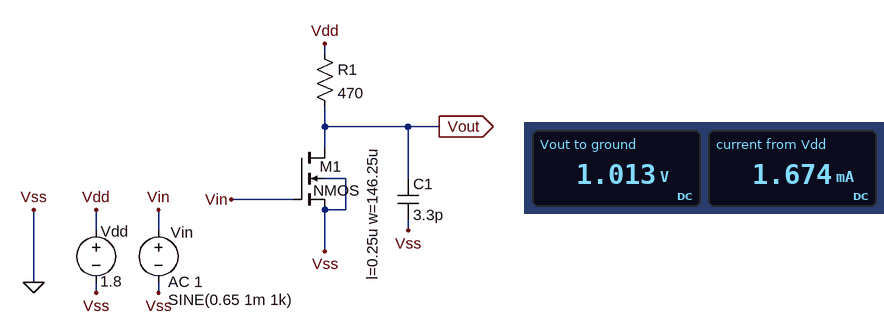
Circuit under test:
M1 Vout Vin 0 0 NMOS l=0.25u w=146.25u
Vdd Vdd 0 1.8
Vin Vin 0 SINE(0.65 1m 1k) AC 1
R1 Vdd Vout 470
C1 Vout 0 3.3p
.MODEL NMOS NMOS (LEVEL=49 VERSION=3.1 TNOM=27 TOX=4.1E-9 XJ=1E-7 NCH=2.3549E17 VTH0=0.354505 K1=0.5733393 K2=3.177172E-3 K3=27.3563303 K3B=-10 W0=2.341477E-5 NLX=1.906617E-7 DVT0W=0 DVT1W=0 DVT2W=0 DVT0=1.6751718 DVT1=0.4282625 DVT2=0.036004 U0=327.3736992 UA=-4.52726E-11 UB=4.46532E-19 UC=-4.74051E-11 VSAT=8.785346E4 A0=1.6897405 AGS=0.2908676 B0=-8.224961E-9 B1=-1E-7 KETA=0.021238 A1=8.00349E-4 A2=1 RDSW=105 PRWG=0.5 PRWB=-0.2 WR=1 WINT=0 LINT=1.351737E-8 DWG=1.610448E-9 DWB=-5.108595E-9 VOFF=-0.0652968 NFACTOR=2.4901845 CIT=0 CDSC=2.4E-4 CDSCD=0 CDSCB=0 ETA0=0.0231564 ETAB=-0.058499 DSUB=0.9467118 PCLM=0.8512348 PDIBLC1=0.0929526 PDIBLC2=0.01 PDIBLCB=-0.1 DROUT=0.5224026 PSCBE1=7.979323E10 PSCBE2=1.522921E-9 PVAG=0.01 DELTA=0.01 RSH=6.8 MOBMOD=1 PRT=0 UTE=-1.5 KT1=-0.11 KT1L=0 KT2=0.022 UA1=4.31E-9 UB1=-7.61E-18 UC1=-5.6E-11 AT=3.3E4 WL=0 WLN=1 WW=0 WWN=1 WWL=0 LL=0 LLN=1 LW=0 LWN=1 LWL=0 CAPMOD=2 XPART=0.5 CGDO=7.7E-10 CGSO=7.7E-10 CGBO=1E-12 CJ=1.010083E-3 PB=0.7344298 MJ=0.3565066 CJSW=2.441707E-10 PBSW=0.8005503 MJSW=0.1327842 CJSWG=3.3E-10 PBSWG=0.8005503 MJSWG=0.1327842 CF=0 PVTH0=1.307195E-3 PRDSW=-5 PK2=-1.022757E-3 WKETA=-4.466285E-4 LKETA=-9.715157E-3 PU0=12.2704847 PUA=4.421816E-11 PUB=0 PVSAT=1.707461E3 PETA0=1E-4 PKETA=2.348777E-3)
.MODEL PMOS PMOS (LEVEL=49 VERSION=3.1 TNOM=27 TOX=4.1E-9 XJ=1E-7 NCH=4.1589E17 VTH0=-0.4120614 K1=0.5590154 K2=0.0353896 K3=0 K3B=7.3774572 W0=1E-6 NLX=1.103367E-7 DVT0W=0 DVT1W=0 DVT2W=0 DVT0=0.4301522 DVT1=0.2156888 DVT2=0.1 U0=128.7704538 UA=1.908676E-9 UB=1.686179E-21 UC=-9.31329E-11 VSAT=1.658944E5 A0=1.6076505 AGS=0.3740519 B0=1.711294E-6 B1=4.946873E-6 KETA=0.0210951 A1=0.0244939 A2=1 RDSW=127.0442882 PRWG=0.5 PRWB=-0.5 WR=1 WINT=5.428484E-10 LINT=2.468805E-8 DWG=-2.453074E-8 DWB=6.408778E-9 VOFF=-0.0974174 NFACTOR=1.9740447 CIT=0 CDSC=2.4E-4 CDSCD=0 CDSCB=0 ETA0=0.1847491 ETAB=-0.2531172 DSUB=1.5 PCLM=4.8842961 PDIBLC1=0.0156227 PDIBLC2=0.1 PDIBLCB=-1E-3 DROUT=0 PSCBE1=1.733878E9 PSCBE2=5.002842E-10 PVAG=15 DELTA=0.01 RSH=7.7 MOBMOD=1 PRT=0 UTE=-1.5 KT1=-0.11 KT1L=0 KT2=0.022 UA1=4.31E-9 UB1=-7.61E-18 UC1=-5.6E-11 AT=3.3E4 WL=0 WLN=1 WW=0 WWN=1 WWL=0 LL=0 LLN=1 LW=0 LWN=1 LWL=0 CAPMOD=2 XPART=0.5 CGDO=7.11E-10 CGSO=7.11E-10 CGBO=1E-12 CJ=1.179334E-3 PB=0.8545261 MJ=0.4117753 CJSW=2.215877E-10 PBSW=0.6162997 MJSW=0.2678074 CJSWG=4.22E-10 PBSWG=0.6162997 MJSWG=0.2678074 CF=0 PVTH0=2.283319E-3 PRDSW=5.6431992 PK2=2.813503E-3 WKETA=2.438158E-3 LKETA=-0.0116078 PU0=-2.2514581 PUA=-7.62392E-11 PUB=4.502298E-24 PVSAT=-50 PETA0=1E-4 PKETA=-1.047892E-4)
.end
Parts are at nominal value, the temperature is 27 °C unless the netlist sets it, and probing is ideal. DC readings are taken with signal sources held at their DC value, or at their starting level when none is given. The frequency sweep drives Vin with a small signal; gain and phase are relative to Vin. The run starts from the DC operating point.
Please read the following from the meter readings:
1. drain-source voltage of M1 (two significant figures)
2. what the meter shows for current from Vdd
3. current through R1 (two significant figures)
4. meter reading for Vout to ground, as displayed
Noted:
1.0 V
1.674 mA
1.7 mA
1.013 V
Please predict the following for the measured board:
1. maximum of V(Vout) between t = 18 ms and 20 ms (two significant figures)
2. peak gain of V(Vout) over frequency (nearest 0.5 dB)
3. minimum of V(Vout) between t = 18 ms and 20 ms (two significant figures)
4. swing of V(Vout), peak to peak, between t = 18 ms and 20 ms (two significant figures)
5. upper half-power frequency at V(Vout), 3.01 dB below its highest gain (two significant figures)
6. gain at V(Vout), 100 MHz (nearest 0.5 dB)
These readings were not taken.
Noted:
1.0 V
18.0 dB
1.0 V
16 mV
110 MHz
15.5 dB
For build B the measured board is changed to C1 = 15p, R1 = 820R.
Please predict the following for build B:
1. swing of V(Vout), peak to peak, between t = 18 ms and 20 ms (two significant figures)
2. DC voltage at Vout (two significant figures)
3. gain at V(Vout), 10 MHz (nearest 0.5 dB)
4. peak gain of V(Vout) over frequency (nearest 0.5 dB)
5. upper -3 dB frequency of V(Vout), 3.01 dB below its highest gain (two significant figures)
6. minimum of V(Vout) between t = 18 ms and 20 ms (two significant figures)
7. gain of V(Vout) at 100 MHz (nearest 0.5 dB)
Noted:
24 mV
530 mV
20.0 dB
21.5 dB
16 MHz
520 mV
5.5 dB
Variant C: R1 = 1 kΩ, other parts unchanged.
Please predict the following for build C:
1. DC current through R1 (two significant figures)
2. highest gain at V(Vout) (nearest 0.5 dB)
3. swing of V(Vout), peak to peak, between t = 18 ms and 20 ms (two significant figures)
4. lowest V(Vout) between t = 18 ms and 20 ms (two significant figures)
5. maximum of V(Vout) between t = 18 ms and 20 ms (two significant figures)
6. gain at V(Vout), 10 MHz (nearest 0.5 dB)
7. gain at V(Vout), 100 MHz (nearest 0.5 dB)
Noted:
1.5 mA
22.0 dB
25 mV
310 mV
340 mV
21.5 dB
16.5 dB
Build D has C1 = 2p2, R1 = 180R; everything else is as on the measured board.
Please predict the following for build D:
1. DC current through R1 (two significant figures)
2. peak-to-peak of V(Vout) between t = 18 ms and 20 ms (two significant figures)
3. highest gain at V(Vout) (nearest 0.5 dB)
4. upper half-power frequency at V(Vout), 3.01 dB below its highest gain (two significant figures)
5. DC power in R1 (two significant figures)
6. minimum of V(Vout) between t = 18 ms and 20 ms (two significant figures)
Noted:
1.8 mA
6.8 mV
10.5 dB
390 MHz
580 µW
1.5 V
